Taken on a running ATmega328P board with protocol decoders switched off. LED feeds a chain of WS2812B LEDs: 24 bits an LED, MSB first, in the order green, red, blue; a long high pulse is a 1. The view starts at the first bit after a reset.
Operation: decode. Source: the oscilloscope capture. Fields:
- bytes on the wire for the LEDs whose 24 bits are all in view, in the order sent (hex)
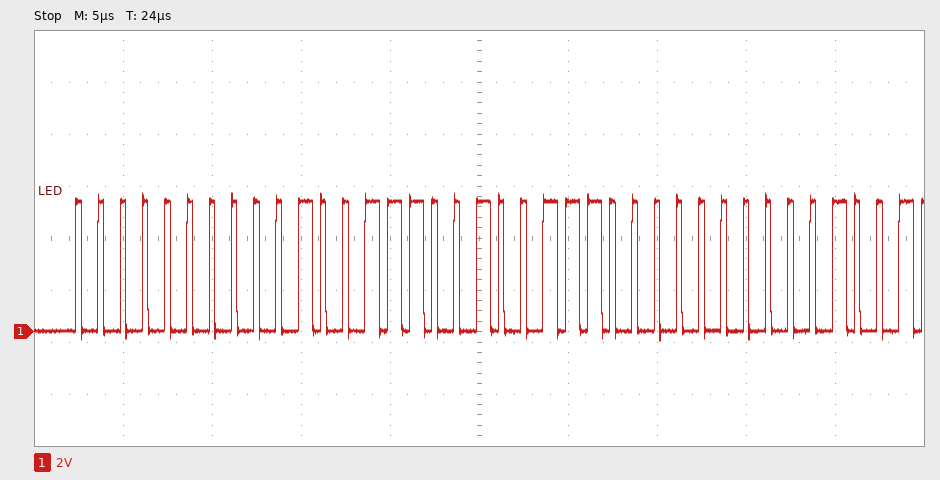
00 27 27
